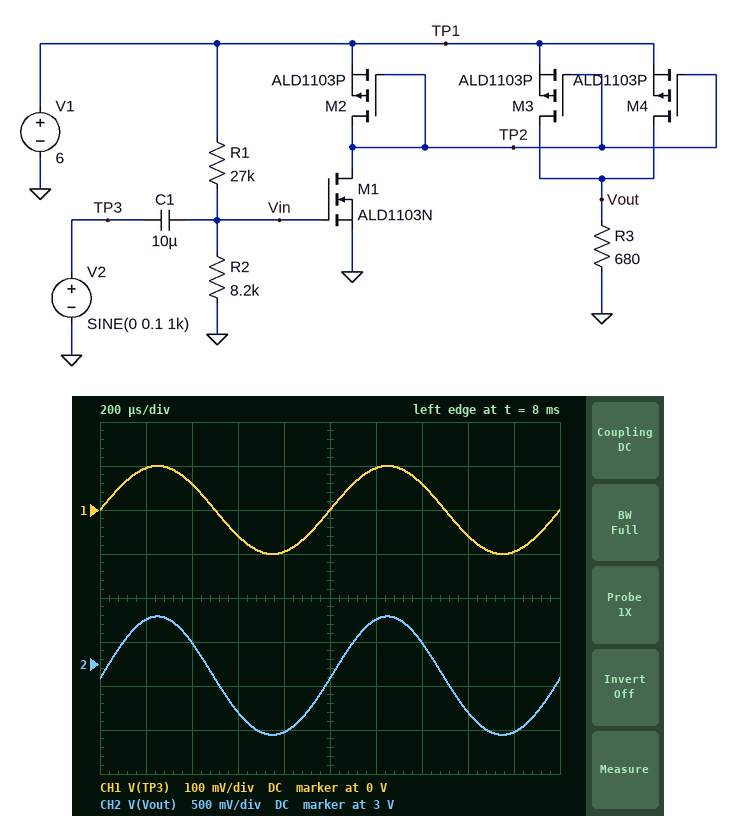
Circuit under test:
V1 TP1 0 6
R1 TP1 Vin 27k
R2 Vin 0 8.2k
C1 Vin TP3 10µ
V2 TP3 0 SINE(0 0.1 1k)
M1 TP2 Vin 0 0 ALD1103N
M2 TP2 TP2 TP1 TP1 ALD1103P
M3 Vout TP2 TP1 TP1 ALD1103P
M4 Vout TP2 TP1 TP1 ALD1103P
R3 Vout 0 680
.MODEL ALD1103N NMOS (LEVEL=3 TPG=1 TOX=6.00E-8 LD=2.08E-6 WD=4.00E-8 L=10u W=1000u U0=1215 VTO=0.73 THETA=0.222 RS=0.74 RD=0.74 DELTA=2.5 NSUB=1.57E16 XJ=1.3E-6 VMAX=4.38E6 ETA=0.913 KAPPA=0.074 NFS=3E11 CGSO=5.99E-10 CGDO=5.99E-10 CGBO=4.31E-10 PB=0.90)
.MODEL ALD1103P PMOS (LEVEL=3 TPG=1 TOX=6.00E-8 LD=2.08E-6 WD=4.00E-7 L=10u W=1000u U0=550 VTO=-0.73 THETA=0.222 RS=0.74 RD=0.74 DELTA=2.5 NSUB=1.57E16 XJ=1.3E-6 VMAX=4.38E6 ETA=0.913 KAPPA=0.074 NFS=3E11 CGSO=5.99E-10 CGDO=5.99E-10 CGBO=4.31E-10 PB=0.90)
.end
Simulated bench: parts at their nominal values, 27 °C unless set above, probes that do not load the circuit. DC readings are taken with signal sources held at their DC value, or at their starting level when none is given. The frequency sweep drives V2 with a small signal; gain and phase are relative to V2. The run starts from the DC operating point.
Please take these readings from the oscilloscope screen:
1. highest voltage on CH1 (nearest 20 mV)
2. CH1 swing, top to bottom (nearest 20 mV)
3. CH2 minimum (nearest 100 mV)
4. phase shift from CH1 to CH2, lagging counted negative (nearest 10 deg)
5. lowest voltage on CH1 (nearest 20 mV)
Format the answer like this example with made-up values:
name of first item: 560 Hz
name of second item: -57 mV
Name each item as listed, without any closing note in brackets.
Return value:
highest voltage on CH1: 100 mV
CH1 swing, top to bottom: 200 mV
CH2 minimum: 2.2 V
phase shift from CH1 to CH2, lagging counted negative: 0 deg
lowest voltage on CH1: -100 mV
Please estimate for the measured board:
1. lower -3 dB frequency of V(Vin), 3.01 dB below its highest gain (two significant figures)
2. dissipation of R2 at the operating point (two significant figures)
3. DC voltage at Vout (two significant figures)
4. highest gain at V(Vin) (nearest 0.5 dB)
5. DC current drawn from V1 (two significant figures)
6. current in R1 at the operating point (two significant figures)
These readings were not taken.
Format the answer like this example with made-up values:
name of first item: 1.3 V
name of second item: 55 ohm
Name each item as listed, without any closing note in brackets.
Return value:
lower -3 dB frequency of V(Vin), 3.01 dB below its highest gain: 2.5 Hz
dissipation of R2 at the operating point: 240 µW
DC voltage at Vout: 2.8 V
highest gain at V(Vin): 0 dB
DC current drawn from V1: 6.4 mA
current in R1 at the operating point: 170 µA
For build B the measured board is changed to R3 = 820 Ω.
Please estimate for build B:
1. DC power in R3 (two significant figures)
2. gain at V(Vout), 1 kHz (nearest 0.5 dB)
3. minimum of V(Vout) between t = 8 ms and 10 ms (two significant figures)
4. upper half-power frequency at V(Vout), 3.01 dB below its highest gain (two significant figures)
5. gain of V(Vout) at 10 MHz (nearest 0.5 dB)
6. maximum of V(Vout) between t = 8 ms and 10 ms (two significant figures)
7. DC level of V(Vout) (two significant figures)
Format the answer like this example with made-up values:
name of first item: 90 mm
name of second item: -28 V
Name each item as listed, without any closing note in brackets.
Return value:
DC power in R3: 14 mW
gain at V(Vout), 1 kHz: 18.0 dB
minimum of V(Vout) between t = 8 ms and 10 ms: 2.6 V
upper half-power frequency at V(Vout), 3.01 dB below its highest gain: 29 MHz
gain of V(Vout) at 10 MHz: 17.5 dB
maximum of V(Vout) between t = 8 ms and 10 ms: 4.2 V
DC level of V(Vout): 3.4 V
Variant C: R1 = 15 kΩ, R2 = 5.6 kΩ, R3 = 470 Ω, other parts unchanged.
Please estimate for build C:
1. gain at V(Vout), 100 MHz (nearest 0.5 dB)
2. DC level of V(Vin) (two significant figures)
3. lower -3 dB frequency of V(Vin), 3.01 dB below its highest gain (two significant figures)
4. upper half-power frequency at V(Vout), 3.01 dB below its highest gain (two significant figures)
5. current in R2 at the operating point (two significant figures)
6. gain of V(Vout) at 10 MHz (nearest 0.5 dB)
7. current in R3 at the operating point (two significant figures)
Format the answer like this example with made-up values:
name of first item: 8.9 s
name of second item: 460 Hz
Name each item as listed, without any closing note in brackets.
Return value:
gain at V(Vout), 100 MHz: 6.5 dB
DC level of V(Vin): 1.6 V
lower -3 dB frequency of V(Vin), 3.01 dB below its highest gain: 3.9 Hz
upper half-power frequency at V(Vout), 3.01 dB below its highest gain: 41 MHz
current in R2 at the operating point: 290 µA
gain of V(Vout) at 10 MHz: 15.0 dB
current in R3 at the operating point: 6.8 mA
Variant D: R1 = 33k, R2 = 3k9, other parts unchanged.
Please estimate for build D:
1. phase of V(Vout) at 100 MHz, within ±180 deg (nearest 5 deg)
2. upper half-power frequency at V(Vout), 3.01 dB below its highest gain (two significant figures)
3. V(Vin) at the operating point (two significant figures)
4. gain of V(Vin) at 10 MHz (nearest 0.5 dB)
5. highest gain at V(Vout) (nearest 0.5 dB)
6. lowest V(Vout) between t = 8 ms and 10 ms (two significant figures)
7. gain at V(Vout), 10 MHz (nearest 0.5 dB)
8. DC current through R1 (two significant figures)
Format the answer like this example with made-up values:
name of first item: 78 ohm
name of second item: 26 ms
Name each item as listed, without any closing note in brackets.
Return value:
phase of V(Vout) at 100 MHz, within ±180 deg: 115 deg
upper half-power frequency at V(Vout), 3.01 dB below its highest gain: 1.2 MHz
V(Vin) at the operating point: 630 mV
gain of V(Vin) at 10 MHz: 0 dB
highest gain at V(Vout): -9.0 dB
lowest V(Vout) between t = 8 ms and 10 ms: 2.7 mV
gain at V(Vout), 10 MHz: -26.0 dB
DC current through R1: 160 µA
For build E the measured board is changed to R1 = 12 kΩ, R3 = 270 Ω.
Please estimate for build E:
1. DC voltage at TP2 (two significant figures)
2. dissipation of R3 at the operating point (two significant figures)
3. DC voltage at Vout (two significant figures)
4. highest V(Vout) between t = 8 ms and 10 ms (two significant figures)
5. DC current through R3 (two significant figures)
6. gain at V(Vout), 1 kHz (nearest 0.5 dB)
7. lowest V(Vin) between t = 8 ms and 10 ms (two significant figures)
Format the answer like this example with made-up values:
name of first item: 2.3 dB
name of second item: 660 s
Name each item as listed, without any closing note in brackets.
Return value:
DC voltage at TP2: 2.5 V
dissipation of R3 at the operating point: 79 mW
DC voltage at Vout: 4.6 V
highest V(Vout) between t = 8 ms and 10 ms: 4.7 V
DC current through R3: 17 mA
gain at V(Vout), 1 kHz: 1.0 dB
lowest V(Vin) between t = 8 ms and 10 ms: 2.3 V
